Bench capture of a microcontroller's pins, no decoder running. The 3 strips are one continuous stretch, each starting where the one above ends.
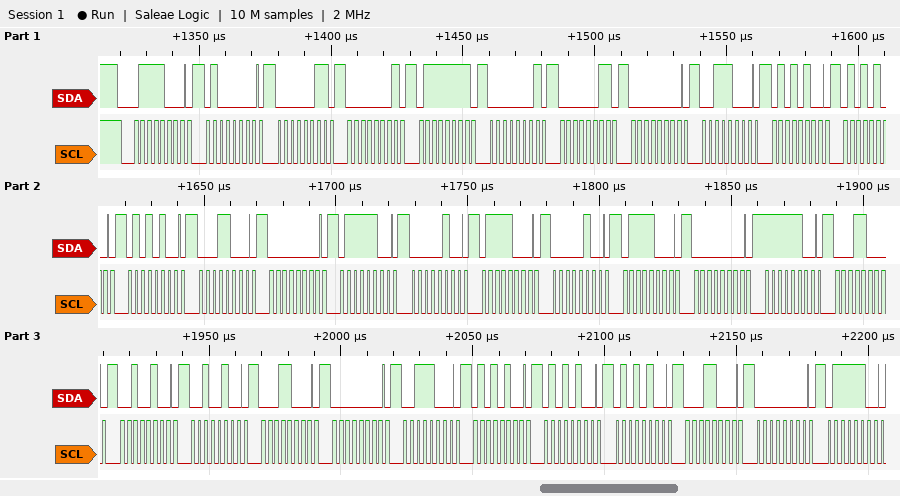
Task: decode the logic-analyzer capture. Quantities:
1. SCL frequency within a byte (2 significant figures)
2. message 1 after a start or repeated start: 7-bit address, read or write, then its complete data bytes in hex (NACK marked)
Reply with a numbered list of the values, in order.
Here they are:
1. 400 kHz
2. 0x3C write: 40 03 01 7F 01 03 00 38 54 54 54 18 00 7C 04 78 04 78 00 FC 18 24 24 18 00 38 54 54 54 18 00 7C
